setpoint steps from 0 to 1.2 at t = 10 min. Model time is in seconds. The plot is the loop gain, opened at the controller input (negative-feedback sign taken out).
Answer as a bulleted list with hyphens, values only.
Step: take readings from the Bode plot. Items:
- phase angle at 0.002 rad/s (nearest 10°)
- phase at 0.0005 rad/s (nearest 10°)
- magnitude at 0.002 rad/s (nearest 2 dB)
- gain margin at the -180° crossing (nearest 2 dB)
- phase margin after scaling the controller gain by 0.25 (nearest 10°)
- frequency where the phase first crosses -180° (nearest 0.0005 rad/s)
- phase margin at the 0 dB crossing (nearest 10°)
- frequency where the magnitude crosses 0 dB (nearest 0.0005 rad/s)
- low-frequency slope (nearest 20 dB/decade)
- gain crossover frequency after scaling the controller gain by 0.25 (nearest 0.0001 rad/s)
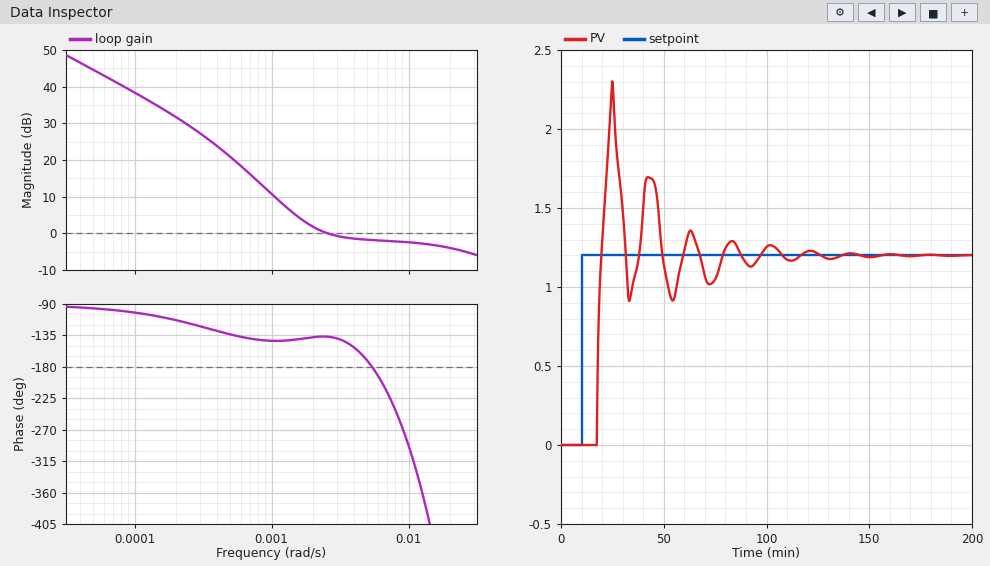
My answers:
- -140°
- -130°
- 2 dB
- 2 dB
- 40°
- 0.0055 rad/s
- 40°
- 0.0025 rad/s
- -20 dB/decade
- 0.0009 rad/s
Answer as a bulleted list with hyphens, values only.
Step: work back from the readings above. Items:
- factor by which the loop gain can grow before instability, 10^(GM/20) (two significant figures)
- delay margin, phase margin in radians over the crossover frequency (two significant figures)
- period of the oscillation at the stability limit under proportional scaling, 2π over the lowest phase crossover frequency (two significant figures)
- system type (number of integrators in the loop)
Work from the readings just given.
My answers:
- 1.3
- 280 s
- 1100 s
- 1
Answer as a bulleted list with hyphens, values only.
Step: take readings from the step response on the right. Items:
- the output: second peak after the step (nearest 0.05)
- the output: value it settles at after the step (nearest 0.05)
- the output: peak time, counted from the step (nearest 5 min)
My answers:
- 1.70
- 1.20
- 15 min
